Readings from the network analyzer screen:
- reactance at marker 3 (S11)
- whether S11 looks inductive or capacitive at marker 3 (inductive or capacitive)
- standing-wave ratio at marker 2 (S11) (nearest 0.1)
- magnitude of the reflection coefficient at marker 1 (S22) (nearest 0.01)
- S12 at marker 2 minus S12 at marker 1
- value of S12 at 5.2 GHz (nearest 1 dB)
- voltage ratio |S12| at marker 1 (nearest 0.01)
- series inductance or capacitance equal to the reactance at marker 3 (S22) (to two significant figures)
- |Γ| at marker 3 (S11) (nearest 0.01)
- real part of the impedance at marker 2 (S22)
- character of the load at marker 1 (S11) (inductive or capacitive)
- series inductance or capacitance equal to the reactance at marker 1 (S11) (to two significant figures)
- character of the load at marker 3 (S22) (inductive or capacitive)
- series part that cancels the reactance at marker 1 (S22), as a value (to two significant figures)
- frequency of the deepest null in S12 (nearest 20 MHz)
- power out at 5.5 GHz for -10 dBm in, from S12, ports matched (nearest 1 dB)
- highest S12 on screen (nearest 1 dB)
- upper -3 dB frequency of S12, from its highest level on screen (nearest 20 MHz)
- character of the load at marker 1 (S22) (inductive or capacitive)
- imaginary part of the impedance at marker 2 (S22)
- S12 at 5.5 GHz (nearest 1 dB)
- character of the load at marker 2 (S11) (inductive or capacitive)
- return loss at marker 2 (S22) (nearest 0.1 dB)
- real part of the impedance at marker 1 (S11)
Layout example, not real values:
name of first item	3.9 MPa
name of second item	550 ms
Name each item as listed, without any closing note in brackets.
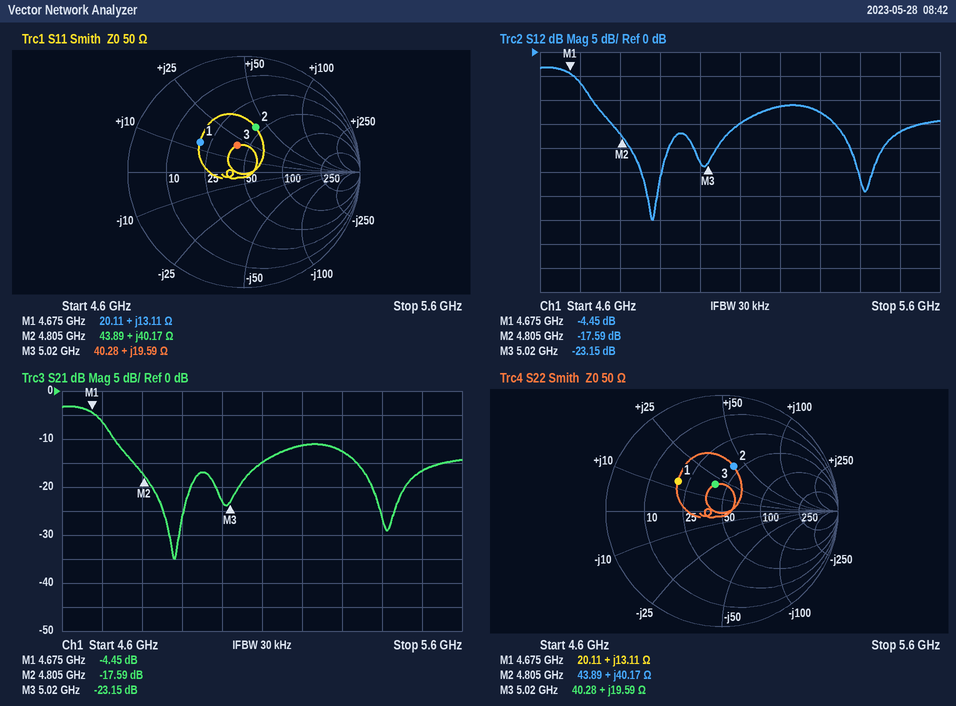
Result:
reactance at marker 3	+19.59 Ω
whether S11 looks inductive or capacitive at marker 3	inductive
standing-wave ratio at marker 2 (S11)	2.3
magnitude of the reflection coefficient at marker 1 (S22)	0.46
S12 at marker 2 minus S12 at marker 1	-13.14 dB
value of S12 at 5.2 GHz	-11 dB
voltage ratio |S12| at marker 1	0.60
series inductance or capacitance equal to the reactance at marker 3 (S22)	620 pH
|Γ| at marker 3 (S11)	0.24
real part of the impedance at marker 2	43.89 Ω
character of the load at marker 1 (S11)	inductive
series inductance or capacitance equal to the reactance at marker 1 (S11)	450 pH
character of the load at marker 3 (S22)	inductive
series part that cancels the reactance at marker 1 (S22), as a value	2.6 pF
frequency of the deepest null in S12	4.88 GHz
power out at 5.5 GHz for -10 dBm in, from S12, ports matched	-27 dBm
highest S12 on screen	-3 dB
upper -3 dB frequency of S12, from its highest level on screen	4.70 GHz
character of the load at marker 1 (S22)	inductive
imaginary part of the impedance at marker 2	+40.17 Ω
S12 at 5.5 GHz	-17 dB
character of the load at marker 2 (S11)	inductive
return loss at marker 2 (S22)	8.0 dB
real part of the impedance at marker 1	20.11 Ω
